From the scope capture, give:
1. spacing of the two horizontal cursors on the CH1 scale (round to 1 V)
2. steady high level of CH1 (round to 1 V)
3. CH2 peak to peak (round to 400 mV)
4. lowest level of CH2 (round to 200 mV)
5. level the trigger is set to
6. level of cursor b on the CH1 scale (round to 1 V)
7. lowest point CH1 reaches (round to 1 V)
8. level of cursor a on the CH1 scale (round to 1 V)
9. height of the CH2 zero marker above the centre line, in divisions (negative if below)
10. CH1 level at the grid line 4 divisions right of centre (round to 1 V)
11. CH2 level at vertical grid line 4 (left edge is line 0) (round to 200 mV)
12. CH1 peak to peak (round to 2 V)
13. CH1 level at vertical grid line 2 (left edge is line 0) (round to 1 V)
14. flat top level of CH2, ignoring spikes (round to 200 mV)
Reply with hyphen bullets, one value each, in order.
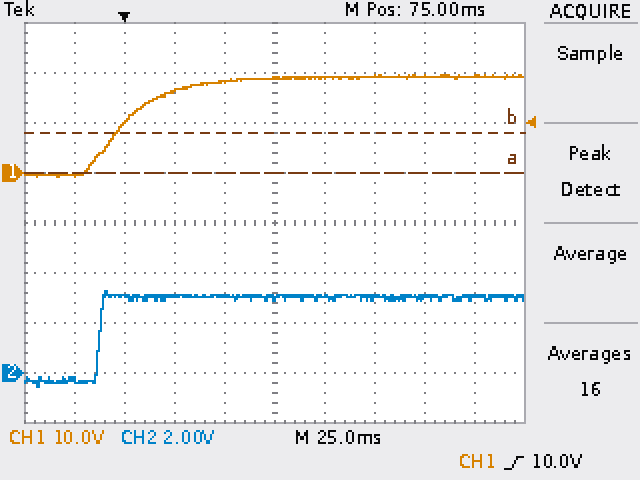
- 8 V
- 19 V
- 4.0 V
- -600 mV
- 10.0 V
- 8 V
- -1 V
- 0 V
- -3.0 div
- 19 V
- 3.0 V
- 20 V
- 10 V
- 3.0 V
